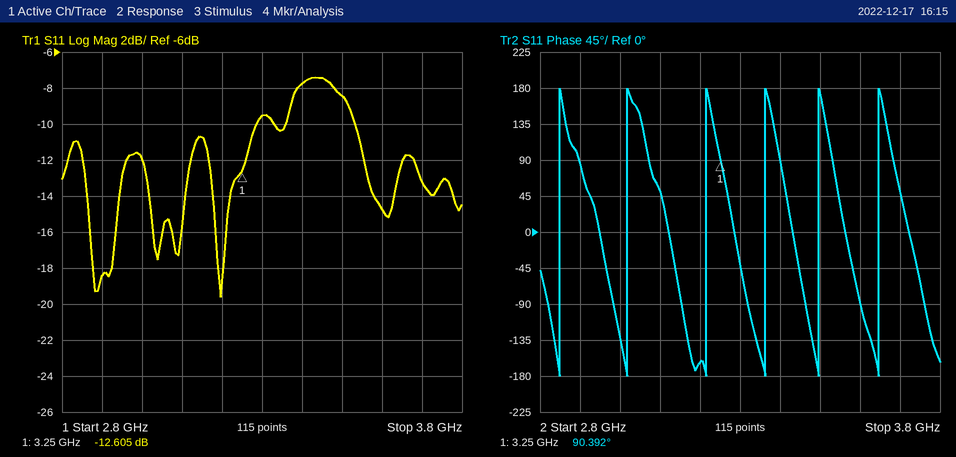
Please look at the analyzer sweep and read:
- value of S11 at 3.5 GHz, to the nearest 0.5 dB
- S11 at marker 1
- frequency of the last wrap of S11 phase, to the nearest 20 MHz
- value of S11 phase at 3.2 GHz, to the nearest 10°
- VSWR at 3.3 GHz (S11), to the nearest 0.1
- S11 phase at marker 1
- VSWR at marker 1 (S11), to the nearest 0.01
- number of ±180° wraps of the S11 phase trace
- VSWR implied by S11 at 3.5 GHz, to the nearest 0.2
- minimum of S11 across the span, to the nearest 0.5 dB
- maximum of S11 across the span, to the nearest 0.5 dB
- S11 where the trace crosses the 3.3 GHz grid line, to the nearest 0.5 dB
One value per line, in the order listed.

-8.5 dB
-12.605 dB
3.64 GHz
-160°
2.0
90.392°
1.61
6
2.2
-19.5 dB
-7.5 dB
-9.5 dB
